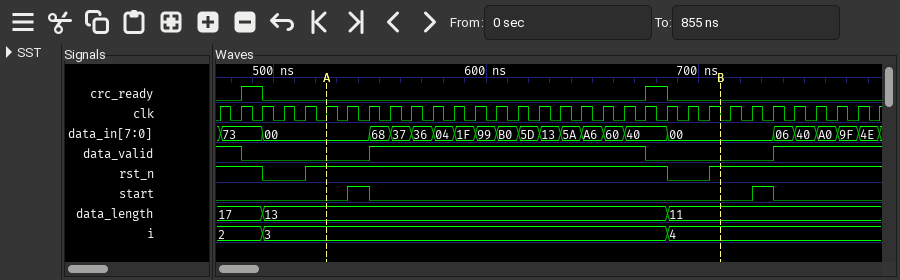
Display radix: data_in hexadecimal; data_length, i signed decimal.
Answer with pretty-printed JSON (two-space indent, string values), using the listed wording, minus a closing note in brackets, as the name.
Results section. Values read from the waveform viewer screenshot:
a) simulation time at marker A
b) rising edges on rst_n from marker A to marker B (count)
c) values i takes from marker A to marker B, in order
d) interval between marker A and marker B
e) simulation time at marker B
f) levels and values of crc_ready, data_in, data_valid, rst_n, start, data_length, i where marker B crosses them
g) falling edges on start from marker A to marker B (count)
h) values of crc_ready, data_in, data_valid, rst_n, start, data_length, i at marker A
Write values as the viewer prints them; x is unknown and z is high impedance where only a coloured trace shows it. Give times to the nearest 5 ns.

{
  "simulation time at marker A": "525 ns",
  "rising edges on rst_n from marker A to marker B": "1",
  "values i takes from marker A to marker B, in order": "3, 4",
  "interval between marker A and marker B": "185 ns",
  "simulation time at marker B": "710 ns",
  "levels and values of crc_ready, data_in, data_valid, rst_n, start, data_length, i where marker B crosses them": "crc_ready=0, data_in=00, data_valid=0, rst_n=1, start=0, data_length=11, i=4",
  "falling edges on start from marker A to marker B": "1",
  "values of crc_ready, data_in, data_valid, rst_n, start, data_length, i at marker A": "crc_ready=0, data_in=00, data_valid=0, rst_n=1, start=0, data_length=13, i=3"
}
